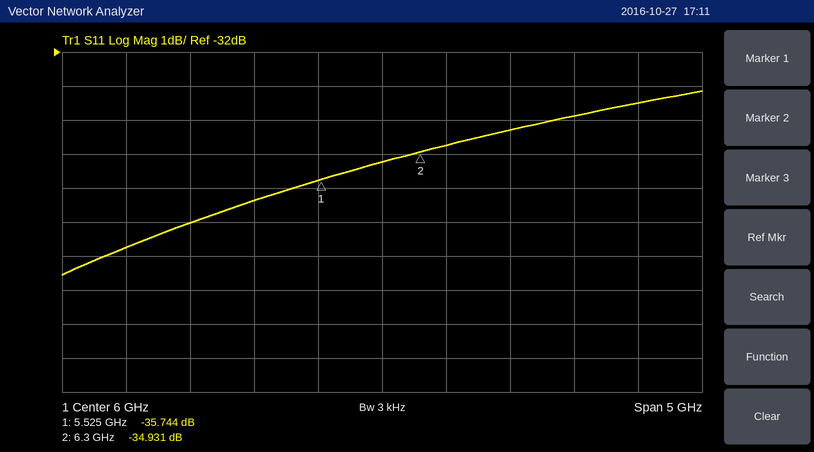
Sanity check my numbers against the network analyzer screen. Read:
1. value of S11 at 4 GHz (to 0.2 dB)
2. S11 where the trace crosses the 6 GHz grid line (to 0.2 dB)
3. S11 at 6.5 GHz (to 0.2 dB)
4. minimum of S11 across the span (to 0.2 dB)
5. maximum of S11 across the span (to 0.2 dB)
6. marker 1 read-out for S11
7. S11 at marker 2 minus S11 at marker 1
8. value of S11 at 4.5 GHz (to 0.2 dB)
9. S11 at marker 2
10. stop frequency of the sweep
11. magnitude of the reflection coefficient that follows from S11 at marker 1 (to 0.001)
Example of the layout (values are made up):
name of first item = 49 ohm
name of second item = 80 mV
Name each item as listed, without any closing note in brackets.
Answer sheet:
value of S11 at 4 GHz = -37.8 dB
S11 where the trace crosses the 6 GHz grid line = -35.2 dB
S11 at 6.5 GHz = -34.8 dB
minimum of S11 across the span = -38.6 dB
maximum of S11 across the span = -33.2 dB
marker 1 read-out for S11 = -35.744 dB
S11 at marker 2 minus S11 at marker 1 = 0.813 dB
value of S11 at 4.5 GHz = -37.0 dB
S11 at marker 2 = -34.931 dB
stop frequency of the sweep = 8.5 GHz
magnitude of the reflection coefficient that follows from S11 at marker 1 = 0.016
